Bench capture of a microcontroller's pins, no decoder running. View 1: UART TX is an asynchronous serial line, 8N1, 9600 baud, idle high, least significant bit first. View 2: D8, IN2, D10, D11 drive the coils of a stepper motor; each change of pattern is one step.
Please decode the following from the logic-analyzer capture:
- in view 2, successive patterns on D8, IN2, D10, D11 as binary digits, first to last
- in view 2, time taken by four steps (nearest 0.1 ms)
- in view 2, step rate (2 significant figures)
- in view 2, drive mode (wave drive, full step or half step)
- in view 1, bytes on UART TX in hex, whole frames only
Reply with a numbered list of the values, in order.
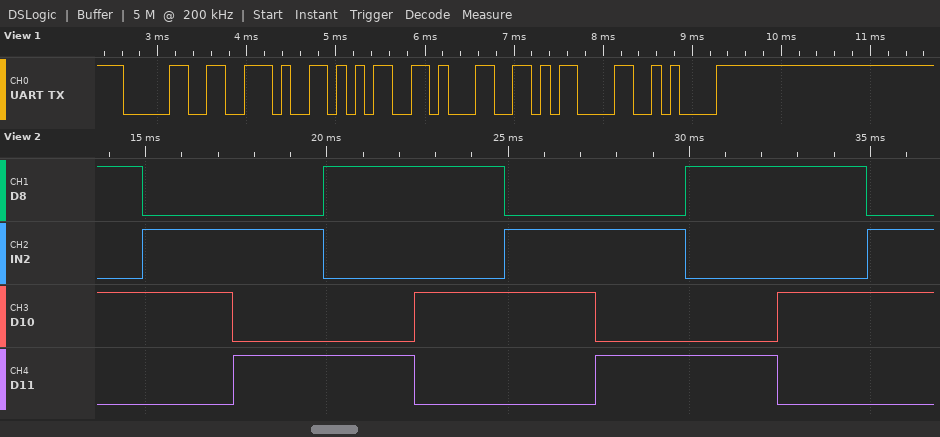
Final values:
1. 1010 0110 0101 1001 1010 0110 0101 1001 1010 0110
2. 10.0 ms
3. 400 steps/s
4. full step
5. 0x30 0x2E 0x35 0x31 0x0D 0x0A
